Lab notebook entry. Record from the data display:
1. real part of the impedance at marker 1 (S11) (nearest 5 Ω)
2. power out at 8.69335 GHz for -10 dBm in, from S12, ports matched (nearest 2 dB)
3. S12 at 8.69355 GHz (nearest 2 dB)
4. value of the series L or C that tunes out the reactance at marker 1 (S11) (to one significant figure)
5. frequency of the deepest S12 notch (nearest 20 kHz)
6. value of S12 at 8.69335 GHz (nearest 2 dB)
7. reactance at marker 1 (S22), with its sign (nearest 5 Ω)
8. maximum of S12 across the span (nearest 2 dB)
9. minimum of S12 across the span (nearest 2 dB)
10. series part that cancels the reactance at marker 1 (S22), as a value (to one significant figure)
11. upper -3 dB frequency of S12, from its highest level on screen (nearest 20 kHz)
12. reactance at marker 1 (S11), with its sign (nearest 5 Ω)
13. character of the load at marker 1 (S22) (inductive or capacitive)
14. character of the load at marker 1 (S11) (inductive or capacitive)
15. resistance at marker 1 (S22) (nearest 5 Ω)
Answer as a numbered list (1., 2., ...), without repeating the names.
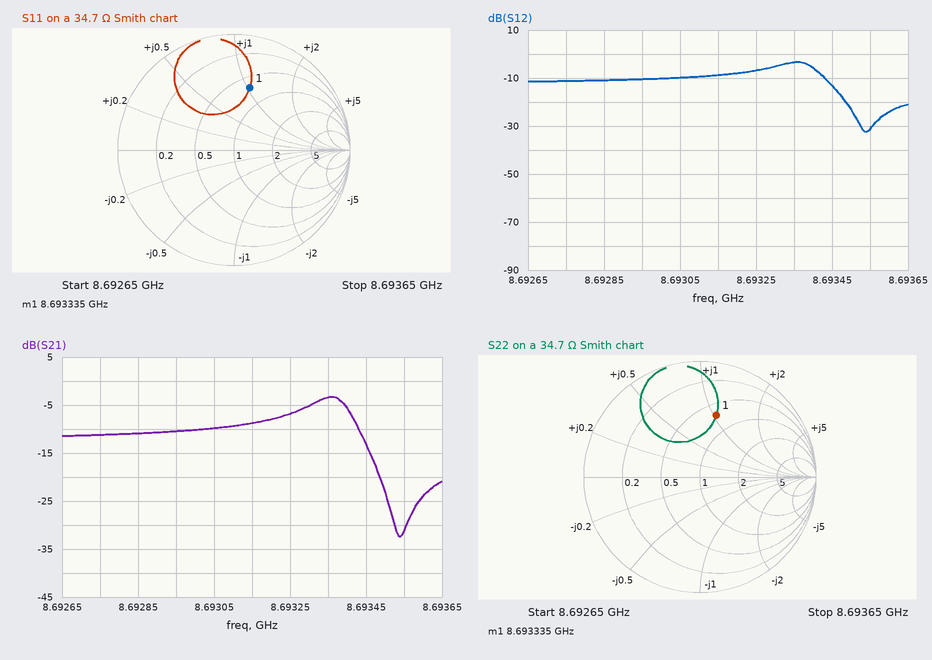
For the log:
1. 25 Ω
2. -14 dBm
3. -32 dB
4. 500 fF
5. 8.69354 GHz
6. -4 dB
7. +35 Ω
8. -4 dB
9. -32 dB
10. 500 fF
11. 8.69340 GHz
12. +35 Ω
13. inductive
14. inductive
15. 25 Ω
